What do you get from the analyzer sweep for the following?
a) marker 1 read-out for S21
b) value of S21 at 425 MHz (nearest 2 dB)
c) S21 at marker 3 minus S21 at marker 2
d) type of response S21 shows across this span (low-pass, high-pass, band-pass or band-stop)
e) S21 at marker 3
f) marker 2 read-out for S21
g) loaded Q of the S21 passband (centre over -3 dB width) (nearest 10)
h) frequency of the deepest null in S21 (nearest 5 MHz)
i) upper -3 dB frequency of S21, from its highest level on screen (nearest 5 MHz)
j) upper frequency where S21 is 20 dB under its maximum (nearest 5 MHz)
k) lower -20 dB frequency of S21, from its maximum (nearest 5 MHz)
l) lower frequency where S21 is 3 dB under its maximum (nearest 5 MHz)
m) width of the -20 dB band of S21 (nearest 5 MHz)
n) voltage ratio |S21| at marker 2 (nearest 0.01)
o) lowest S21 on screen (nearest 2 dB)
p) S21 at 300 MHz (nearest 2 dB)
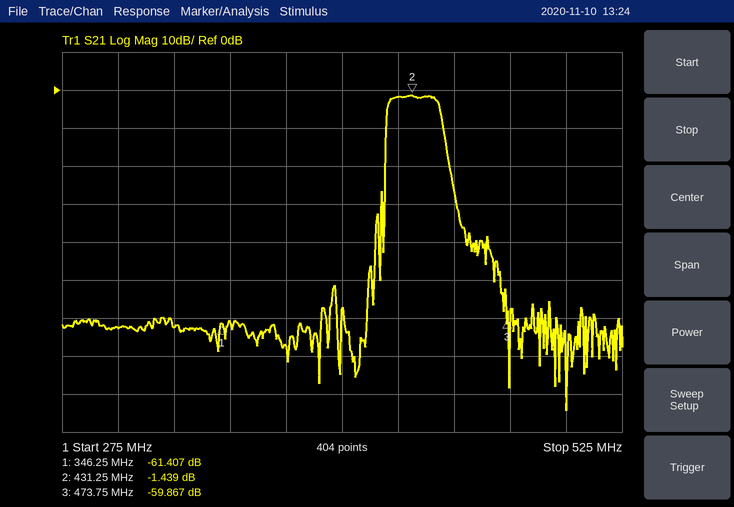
-61.407 dB
-2 dB
-58.428 dB
band-pass
-59.867 dB
-1.439 dB
20
500 MHz
445 MHz
450 MHz
420 MHz
420 MHz
30 MHz
0.85
-84 dB
-62 dB
